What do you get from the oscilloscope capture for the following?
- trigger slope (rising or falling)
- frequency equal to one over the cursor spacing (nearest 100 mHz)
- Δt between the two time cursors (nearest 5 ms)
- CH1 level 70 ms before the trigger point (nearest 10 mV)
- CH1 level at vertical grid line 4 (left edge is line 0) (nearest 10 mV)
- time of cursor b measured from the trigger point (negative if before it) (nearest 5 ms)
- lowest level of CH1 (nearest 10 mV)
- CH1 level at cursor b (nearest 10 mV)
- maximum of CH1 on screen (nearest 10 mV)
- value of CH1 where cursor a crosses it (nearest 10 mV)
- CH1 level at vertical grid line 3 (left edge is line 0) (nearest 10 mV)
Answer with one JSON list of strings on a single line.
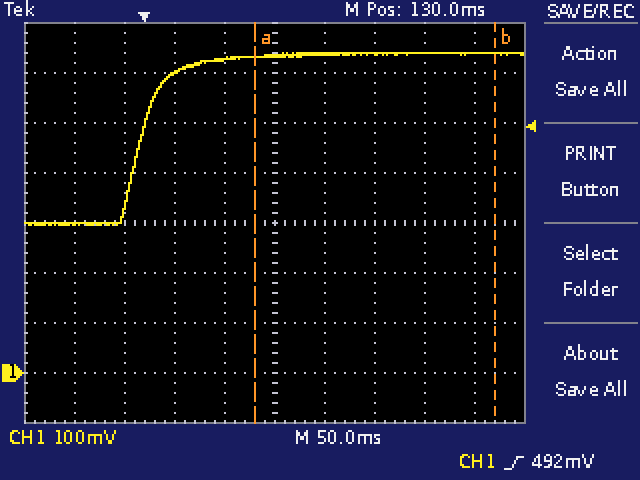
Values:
["rising", "4.2 Hz", "240 ms", "300 mV", "630 mV", "+350 ms", "300 mV", "640 mV", "640 mV", "630 mV", "600 mV"]
